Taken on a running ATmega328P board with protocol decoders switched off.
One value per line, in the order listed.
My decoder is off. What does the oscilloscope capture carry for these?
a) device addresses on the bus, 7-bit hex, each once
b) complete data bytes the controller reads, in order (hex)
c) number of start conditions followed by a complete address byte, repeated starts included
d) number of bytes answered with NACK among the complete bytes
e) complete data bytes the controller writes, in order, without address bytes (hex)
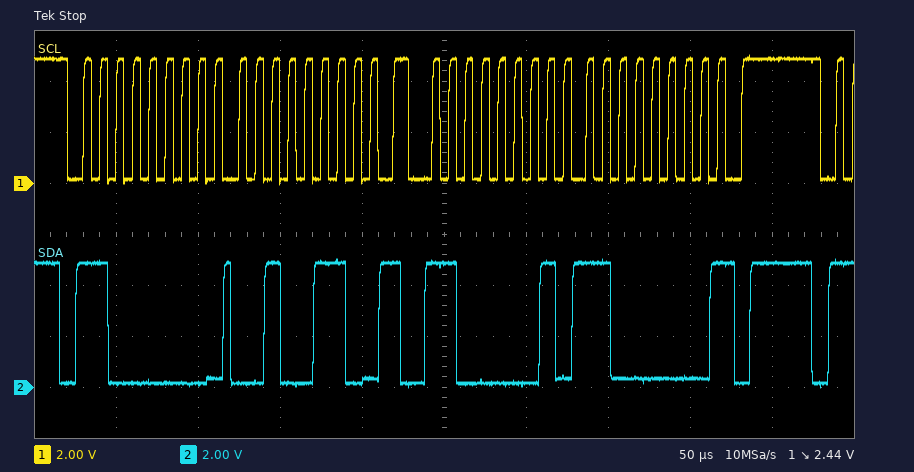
0x60
C0
2
1
26
